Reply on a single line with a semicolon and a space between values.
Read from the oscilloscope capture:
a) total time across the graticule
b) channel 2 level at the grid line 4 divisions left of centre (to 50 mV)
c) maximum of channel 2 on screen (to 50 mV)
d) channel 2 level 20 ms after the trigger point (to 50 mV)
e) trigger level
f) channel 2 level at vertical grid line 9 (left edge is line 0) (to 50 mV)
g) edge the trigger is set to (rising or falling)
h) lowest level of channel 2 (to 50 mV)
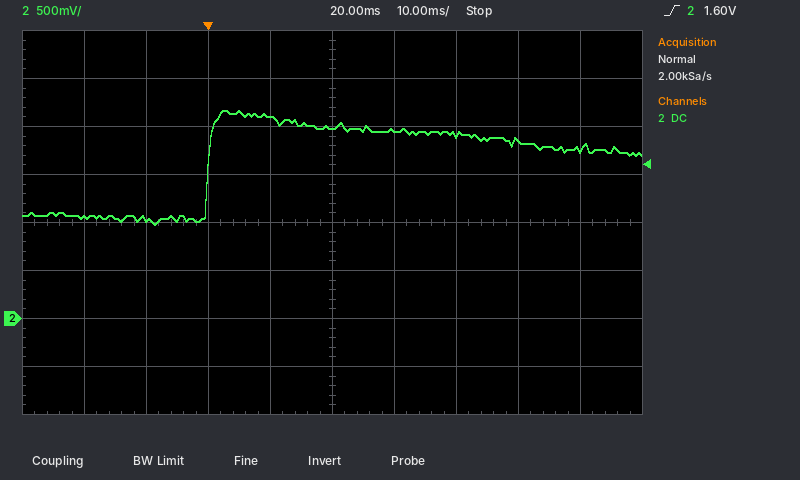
100 ms; 1.05 V; 2.15 V; 2.00 V; 1.60 V; 1.75 V; rising; 1.00 V
